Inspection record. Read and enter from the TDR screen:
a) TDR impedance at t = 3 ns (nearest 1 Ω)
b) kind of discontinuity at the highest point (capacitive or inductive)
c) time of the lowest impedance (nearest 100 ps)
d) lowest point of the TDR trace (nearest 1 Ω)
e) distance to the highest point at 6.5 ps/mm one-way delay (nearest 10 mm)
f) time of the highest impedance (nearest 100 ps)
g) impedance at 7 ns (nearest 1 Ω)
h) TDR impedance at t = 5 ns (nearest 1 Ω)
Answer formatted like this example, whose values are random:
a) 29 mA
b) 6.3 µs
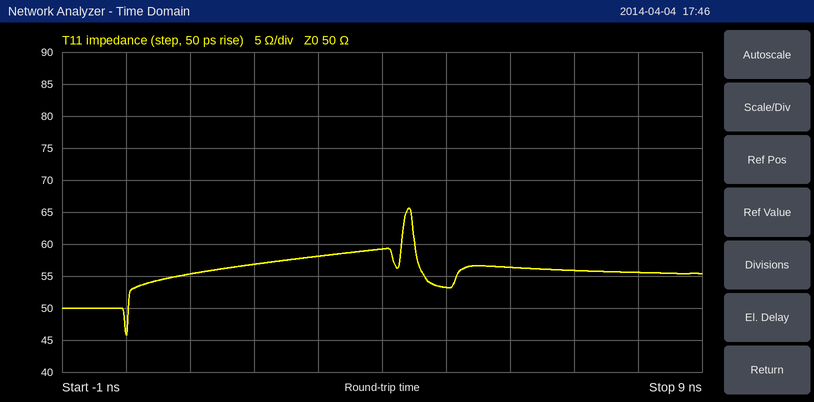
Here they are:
a) 58 Ω
b) inductive
c) 0.0 ns
d) 46 Ω
e) 340 mm
f) 4.4 ns
g) 56 Ω
h) 53 Ω
